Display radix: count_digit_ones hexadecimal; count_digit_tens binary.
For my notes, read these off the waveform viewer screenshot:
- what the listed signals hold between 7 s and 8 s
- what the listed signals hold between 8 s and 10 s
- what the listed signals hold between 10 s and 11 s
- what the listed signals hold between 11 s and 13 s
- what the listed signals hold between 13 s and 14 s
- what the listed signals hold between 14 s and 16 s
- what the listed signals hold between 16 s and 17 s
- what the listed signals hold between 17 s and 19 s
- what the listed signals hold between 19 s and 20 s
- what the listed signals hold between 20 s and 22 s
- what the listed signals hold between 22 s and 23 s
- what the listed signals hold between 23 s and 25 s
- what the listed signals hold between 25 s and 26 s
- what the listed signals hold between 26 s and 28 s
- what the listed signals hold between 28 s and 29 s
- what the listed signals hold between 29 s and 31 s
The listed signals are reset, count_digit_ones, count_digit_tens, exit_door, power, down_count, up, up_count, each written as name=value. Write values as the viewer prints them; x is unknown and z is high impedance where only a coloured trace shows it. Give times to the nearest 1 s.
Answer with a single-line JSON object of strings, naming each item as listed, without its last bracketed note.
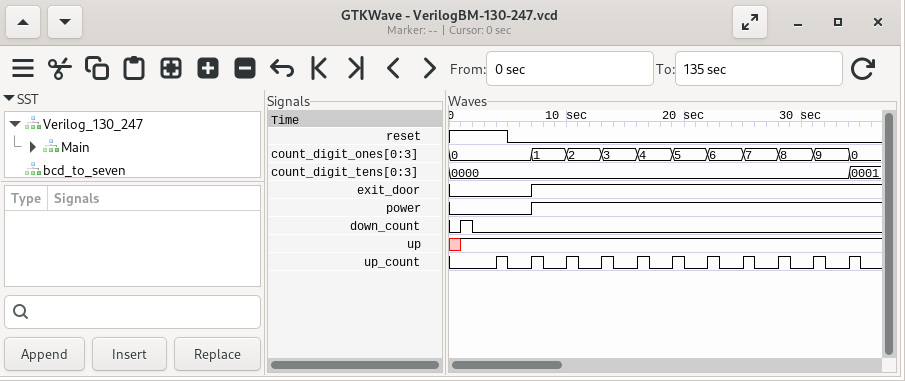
{"what the listed signals hold between 7 s and 8 s": "reset=0, count_digit_ones=1, count_digit_tens=0000, exit_door=1, power=1, down_count=0, up=1, up_count=1", "what the listed signals hold between 8 s and 10 s": "reset=0, count_digit_ones=1, count_digit_tens=0000, exit_door=1, power=1, down_count=0, up=1, up_count=0", "what the listed signals hold between 10 s and 11 s": "reset=0, count_digit_ones=2, count_digit_tens=0000, exit_door=1, power=1, down_count=0, up=1, up_count=1", "what the listed signals hold between 11 s and 13 s": "reset=0, count_digit_ones=2, count_digit_tens=0000, exit_door=1, power=1, down_count=0, up=1, up_count=0", "what the listed signals hold between 13 s and 14 s": "reset=0, count_digit_ones=3, count_digit_tens=0000, exit_door=1, power=1, down_count=0, up=1, up_count=1", "what the listed signals hold between 14 s and 16 s": "reset=0, count_digit_ones=3, count_digit_tens=0000, exit_door=1, power=1, down_count=0, up=1, up_count=0", "what the listed signals hold between 16 s and 17 s": "reset=0, count_digit_ones=4, count_digit_tens=0000, exit_door=1, power=1, down_count=0, up=1, up_count=1", "what the listed signals hold between 17 s and 19 s": "reset=0, count_digit_ones=4, count_digit_tens=0000, exit_door=1, power=1, down_count=0, up=1, up_count=0", "what the listed signals hold between 19 s and 20 s": "reset=0, count_digit_ones=5, count_digit_tens=0000, exit_door=1, power=1, down_count=0, up=1, up_count=1", "what the listed signals hold between 20 s and 22 s": "reset=0, count_digit_ones=5, count_digit_tens=0000, exit_door=1, power=1, down_count=0, up=1, up_count=0", "what the listed signals hold between 22 s and 23 s": "reset=0, count_digit_ones=6, count_digit_tens=0000, exit_door=1, power=1, down_count=0, up=1, up_count=1", "what the listed signals hold between 23 s and 25 s": "reset=0, count_digit_ones=6, count_digit_tens=0000, exit_door=1, power=1, down_count=0, up=1, up_count=0", "what the listed signals hold between 25 s and 26 s": "reset=0, count_digit_ones=7, count_digit_tens=0000, exit_door=1, power=1, down_count=0, up=1, up_count=1", "what the listed signals hold between 26 s and 28 s": "reset=0, count_digit_ones=7, count_digit_tens=0000, exit_door=1, power=1, down_count=0, up=1, up_count=0", "what the listed signals hold between 28 s and 29 s": "reset=0, count_digit_ones=8, count_digit_tens=0000, exit_door=1, power=1, down_count=0, up=1, up_count=1", "what the listed signals hold between 29 s and 31 s": "reset=0, count_digit_ones=8, count_digit_tens=0000, exit_door=1, power=1, down_count=0, up=1, up_count=0"}
